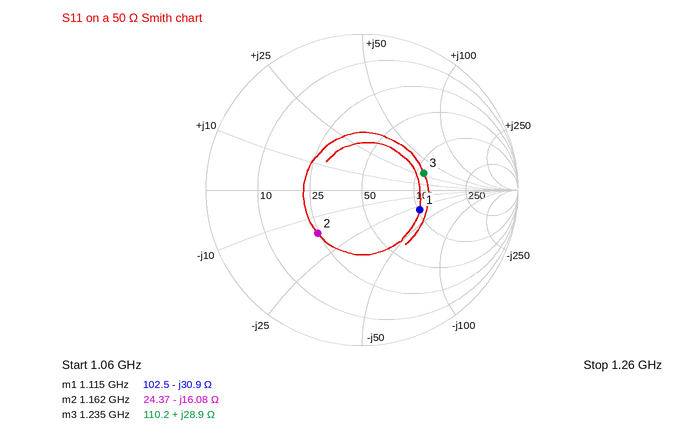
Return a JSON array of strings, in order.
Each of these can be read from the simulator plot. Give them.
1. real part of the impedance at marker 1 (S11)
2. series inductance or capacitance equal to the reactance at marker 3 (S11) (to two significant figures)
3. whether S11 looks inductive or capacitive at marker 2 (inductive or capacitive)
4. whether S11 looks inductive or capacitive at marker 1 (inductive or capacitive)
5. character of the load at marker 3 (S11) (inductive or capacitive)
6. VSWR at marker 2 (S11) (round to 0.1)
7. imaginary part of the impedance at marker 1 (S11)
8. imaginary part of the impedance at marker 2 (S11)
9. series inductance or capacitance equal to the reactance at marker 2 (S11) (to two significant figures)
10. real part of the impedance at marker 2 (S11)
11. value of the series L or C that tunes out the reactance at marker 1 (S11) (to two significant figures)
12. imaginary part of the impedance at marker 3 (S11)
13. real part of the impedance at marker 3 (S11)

["102.5 Ω", "3.7 nH", "capacitive", "capacitive", "inductive", "2.3", "-30.9 Ω", "-16.08 Ω", "8.5 pF", "24.37 Ω", "4.4 nH", "+28.9 Ω", "110.2 Ω"]
